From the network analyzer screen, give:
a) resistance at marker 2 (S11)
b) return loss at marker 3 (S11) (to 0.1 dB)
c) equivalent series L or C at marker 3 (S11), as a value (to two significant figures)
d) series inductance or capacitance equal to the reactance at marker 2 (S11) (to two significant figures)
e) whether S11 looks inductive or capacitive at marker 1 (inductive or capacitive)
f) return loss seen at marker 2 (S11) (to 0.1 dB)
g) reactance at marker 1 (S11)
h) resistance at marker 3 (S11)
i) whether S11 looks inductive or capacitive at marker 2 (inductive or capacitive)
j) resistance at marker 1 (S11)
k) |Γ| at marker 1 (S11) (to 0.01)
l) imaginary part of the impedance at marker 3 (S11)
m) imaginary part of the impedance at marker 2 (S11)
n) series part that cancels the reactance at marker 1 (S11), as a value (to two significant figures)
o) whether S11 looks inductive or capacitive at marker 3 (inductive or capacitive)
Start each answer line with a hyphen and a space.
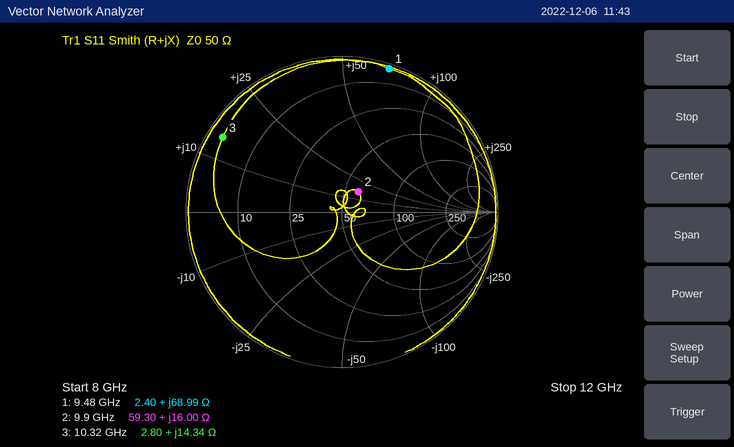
- 59.30 Ω
- 0.9 dB
- 220 pH
- 260 pH
- inductive
- 15.5 dB
- +68.99 Ω
- 2.80 Ω
- inductive
- 2.40 Ω
- 0.97
- +14.34 Ω
- +16.00 Ω
- 240 fF
- inductive
